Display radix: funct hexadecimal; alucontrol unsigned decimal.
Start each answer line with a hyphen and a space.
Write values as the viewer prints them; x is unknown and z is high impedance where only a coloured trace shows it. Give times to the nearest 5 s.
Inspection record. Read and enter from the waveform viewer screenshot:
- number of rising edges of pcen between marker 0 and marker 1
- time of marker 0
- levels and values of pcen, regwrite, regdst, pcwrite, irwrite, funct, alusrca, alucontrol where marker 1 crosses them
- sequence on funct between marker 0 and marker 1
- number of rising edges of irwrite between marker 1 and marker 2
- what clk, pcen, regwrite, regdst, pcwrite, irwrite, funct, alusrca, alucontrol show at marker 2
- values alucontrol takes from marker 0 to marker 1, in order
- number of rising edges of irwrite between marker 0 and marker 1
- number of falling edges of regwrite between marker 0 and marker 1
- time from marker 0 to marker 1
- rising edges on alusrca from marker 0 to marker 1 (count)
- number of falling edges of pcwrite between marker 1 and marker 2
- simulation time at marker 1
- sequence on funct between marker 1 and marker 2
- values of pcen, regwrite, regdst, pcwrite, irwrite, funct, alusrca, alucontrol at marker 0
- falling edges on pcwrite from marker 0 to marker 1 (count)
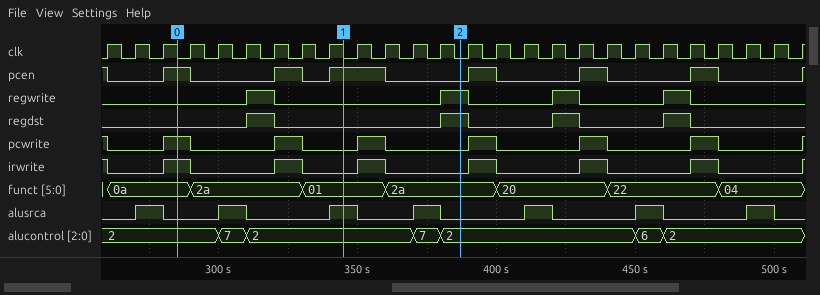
- 2
- 285 s
- pcen=1, regwrite=0, regdst=0, pcwrite=0, irwrite=0, funct=01, alusrca=1, alucontrol=2
- 0a, 2a, 01
- 1
- clk=0, pcen=0, regwrite=1, regdst=1, pcwrite=0, irwrite=0, funct=2a, alusrca=0, alucontrol=2
- 2, 7, 2
- 1
- 1
- 60 s
- 2
- 1
- 345 s
- 01, 2a
- pcen=1, regwrite=0, regdst=0, pcwrite=1, irwrite=1, funct=0a, alusrca=0, alucontrol=2
- 2
